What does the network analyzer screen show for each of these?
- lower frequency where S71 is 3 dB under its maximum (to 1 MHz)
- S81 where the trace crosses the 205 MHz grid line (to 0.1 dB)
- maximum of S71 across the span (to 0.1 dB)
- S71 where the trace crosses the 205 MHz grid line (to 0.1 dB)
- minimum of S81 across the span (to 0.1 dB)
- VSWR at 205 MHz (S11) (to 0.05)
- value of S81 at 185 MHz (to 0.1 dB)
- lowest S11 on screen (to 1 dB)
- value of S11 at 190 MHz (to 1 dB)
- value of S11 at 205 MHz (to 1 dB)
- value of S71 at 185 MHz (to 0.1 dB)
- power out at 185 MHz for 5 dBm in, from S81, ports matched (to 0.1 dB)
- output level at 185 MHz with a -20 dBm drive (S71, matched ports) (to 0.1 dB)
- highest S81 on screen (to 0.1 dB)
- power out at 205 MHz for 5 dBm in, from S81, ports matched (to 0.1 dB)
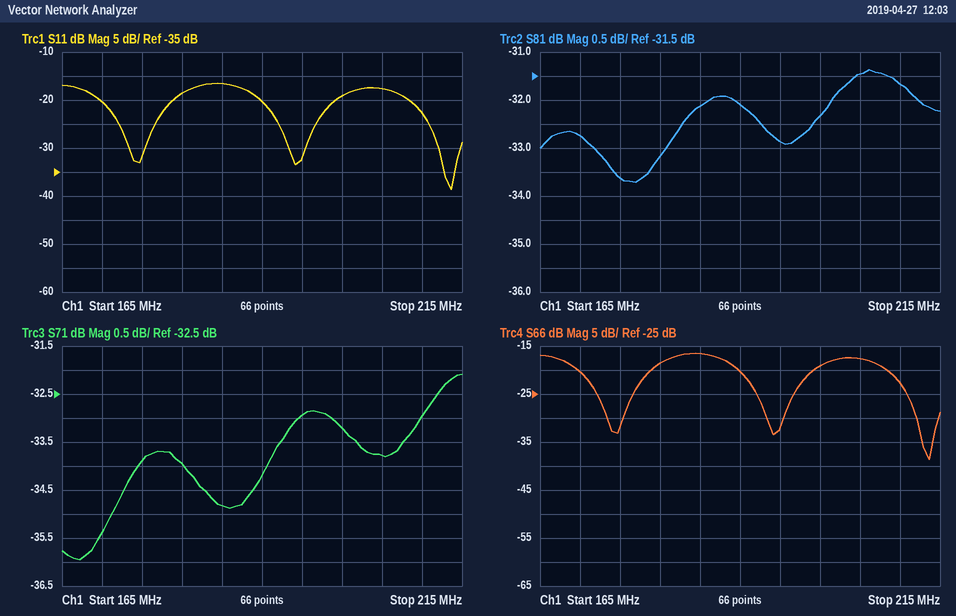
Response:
171 MHz
-31.5 dB
-32.1 dB
-33.8 dB
-33.7 dB
1.30
-32.1 dB
-39 dB
-20 dB
-18 dB
-34.8 dB
-27.1 dBm
-54.8 dBm
-31.4 dB
-26.5 dBm
